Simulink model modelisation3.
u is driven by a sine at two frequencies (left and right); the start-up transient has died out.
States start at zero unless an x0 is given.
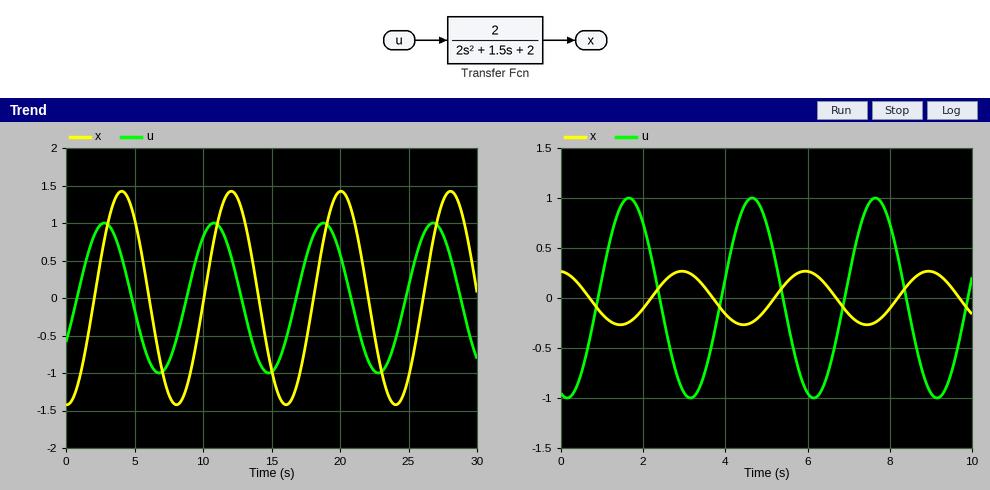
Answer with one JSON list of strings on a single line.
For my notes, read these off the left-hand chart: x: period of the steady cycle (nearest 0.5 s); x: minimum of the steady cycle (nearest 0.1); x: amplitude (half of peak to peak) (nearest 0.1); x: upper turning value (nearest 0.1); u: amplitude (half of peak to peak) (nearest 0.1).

["8.0 s", "-1.4", "1.4", "1.4", "1.0"]
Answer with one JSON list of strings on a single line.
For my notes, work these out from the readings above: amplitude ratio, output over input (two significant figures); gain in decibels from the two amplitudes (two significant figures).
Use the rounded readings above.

["1.4", "2.9 dB"]
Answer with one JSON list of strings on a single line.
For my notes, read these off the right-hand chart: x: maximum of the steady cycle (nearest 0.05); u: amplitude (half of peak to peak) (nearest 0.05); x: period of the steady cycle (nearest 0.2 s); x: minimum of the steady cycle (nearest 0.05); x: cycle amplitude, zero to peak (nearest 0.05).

["0.25", "1.00", "3.0 s", "-0.25", "0.25"]
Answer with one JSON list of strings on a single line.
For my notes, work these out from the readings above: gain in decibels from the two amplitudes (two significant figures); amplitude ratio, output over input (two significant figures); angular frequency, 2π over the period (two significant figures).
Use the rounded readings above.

["-12 dB", "0.25", "2.1 rad/s"]
